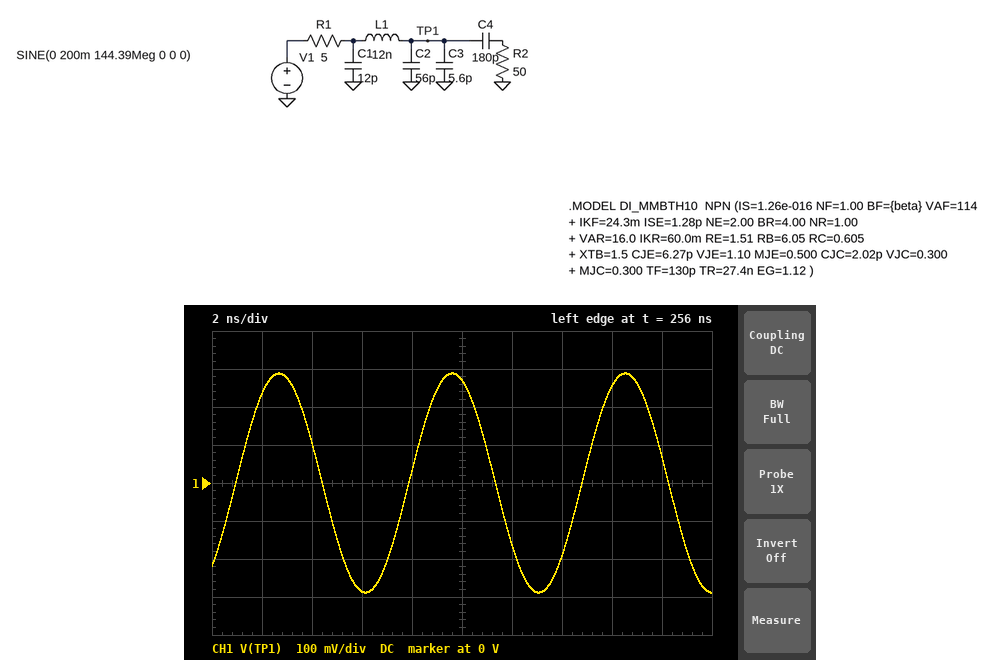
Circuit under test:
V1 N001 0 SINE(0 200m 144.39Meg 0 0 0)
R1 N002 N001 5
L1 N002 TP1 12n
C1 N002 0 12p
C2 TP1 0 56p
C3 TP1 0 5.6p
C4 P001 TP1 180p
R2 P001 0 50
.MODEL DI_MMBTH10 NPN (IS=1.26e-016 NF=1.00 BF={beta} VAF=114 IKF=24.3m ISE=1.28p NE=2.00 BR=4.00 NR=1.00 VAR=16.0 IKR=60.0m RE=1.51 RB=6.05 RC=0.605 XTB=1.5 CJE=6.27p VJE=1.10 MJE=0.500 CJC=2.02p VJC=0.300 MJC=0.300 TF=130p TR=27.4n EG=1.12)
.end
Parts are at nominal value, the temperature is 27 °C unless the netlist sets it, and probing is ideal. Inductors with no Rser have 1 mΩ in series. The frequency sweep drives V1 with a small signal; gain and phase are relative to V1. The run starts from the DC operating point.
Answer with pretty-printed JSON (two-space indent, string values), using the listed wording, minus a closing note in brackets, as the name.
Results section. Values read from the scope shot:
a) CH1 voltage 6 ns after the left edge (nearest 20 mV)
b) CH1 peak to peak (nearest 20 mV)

{
  "CH1 voltage 6 ns after the left edge": "-280 mV",
  "CH1 peak to peak": "580 mV"
}
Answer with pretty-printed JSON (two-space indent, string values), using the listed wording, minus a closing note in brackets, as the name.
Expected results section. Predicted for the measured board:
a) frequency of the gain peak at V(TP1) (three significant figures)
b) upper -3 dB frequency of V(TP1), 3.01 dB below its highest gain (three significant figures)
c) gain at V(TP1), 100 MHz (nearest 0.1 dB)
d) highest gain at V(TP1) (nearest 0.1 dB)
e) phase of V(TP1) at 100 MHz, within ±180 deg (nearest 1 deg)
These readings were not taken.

{
  "frequency of the gain peak at V(TP1)": "175 MHz",
  "upper -3 dB frequency of V(TP1), 3.01 dB below its highest gain": "230 MHz",
  "gain at V(TP1), 100 MHz": "1.3 dB",
  "highest gain at V(TP1)": "3.9 dB",
  "phase of V(TP1) at 100 MHz, within ±180 deg": "-26 deg"
}
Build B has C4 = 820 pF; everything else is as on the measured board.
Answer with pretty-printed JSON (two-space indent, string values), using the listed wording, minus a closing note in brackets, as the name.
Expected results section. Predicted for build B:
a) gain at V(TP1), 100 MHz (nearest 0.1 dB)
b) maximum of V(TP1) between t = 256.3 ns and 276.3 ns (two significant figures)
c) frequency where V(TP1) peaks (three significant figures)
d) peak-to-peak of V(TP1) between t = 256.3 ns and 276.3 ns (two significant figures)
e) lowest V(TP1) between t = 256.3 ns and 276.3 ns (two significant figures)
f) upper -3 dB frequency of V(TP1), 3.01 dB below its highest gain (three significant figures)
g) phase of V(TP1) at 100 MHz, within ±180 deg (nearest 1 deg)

{
  "gain at V(TP1), 100 MHz": "1.1 dB",
  "maximum of V(TP1) between t = 256.3 ns and 276.3 ns": "280 mV",
  "frequency where V(TP1) peaks": "177 MHz",
  "peak-to-peak of V(TP1) between t = 256.3 ns and 276.3 ns": "570 mV",
  "lowest V(TP1) between t = 256.3 ns and 276.3 ns": "-280 mV",
  "upper -3 dB frequency of V(TP1), 3.01 dB below its highest gain": "232 MHz",
  "phase of V(TP1) at 100 MHz, within ±180 deg": "-25 deg"
}
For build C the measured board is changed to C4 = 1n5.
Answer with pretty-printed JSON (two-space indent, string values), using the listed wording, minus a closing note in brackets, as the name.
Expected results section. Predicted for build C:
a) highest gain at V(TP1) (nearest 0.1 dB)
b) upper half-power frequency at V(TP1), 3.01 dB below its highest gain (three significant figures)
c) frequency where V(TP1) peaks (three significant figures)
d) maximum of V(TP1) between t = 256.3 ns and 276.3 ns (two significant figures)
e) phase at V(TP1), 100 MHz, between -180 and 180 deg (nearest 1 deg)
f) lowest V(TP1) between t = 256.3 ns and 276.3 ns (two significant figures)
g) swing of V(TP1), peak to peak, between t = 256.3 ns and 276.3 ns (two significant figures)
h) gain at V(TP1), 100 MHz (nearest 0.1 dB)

{
  "highest gain at V(TP1)": "3.9 dB",
  "upper half-power frequency at V(TP1), 3.01 dB below its highest gain": "232 MHz",
  "frequency where V(TP1) peaks": "177 MHz",
  "maximum of V(TP1) between t = 256.3 ns and 276.3 ns": "280 mV",
  "phase at V(TP1), 100 MHz, between -180 and 180 deg": "-25 deg",
  "lowest V(TP1) between t = 256.3 ns and 276.3 ns": "-280 mV",
  "swing of V(TP1), peak to peak, between t = 256.3 ns and 276.3 ns": "570 mV",
  "gain at V(TP1), 100 MHz": "1.1 dB"
}
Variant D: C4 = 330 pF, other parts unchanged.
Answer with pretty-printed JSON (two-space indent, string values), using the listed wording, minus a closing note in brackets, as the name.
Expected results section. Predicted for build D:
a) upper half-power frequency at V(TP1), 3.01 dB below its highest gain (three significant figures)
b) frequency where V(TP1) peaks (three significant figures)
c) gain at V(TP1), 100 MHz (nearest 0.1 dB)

{
  "upper half-power frequency at V(TP1), 3.01 dB below its highest gain": "231 MHz",
  "frequency where V(TP1) peaks": "176 MHz",
  "gain at V(TP1), 100 MHz": "1.2 dB"
}
